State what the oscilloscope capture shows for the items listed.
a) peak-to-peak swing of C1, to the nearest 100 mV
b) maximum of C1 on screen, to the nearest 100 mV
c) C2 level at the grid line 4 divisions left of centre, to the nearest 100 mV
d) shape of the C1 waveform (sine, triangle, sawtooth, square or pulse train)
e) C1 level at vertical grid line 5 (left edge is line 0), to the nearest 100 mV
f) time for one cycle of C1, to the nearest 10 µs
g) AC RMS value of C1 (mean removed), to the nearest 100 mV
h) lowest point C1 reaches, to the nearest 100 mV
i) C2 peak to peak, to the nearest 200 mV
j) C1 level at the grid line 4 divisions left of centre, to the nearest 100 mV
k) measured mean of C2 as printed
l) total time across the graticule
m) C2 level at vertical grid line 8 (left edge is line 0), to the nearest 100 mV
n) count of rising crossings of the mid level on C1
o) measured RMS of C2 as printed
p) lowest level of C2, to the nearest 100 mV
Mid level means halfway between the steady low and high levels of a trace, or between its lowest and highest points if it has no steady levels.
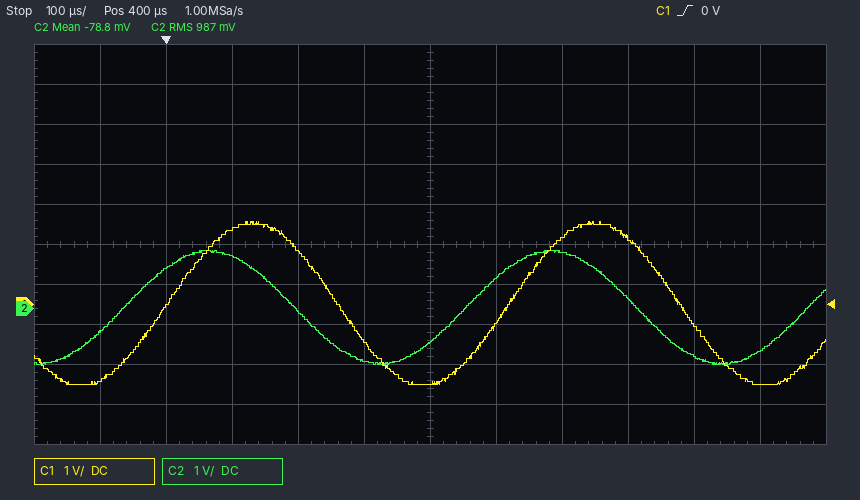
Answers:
4.1 V
2.1 V
1.0 V
sine
-900 mV
520 µs
1.4 V
-2.0 V
2.8 V
0.0 V
-78.8 mV
1.2 ms
1.4 V
2
987 mV
-1.4 V
